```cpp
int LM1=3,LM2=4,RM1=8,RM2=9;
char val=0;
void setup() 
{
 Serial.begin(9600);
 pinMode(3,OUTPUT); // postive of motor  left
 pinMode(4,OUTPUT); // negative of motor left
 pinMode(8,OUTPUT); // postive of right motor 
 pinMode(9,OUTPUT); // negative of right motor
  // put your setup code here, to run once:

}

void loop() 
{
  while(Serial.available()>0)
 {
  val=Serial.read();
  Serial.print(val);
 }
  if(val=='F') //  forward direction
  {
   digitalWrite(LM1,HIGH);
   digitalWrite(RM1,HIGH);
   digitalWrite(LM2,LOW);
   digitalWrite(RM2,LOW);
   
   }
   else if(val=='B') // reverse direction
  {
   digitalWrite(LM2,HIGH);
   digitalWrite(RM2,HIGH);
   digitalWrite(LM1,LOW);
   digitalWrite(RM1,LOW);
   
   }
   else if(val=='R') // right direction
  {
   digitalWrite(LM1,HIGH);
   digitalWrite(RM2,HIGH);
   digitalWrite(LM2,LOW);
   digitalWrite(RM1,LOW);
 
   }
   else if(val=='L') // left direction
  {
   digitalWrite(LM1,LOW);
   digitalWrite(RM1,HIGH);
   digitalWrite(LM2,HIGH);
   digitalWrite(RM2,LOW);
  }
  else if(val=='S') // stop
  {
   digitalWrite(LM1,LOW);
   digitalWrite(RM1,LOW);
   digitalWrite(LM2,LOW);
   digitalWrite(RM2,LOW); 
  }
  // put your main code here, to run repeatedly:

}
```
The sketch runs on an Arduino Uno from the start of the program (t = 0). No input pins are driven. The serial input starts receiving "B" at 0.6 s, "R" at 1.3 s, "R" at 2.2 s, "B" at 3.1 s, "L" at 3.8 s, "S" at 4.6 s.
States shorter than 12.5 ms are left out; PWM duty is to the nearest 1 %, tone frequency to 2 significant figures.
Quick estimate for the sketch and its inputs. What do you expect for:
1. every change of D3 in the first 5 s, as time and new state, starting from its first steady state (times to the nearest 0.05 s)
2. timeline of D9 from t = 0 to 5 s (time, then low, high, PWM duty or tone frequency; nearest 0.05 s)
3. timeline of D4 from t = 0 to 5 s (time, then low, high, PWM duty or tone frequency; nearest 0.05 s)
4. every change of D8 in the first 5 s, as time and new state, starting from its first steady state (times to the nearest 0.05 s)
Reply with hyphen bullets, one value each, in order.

- 0 s low; 1.3 s high; 3.1 s low
- 0 s low; 0.6 s high; 3.8 s low
- 0 s low; 0.6 s high; 1.3 s low; 3.1 s high; 4.6 s low
- 0 s low; 3.8 s high; 4.6 s low
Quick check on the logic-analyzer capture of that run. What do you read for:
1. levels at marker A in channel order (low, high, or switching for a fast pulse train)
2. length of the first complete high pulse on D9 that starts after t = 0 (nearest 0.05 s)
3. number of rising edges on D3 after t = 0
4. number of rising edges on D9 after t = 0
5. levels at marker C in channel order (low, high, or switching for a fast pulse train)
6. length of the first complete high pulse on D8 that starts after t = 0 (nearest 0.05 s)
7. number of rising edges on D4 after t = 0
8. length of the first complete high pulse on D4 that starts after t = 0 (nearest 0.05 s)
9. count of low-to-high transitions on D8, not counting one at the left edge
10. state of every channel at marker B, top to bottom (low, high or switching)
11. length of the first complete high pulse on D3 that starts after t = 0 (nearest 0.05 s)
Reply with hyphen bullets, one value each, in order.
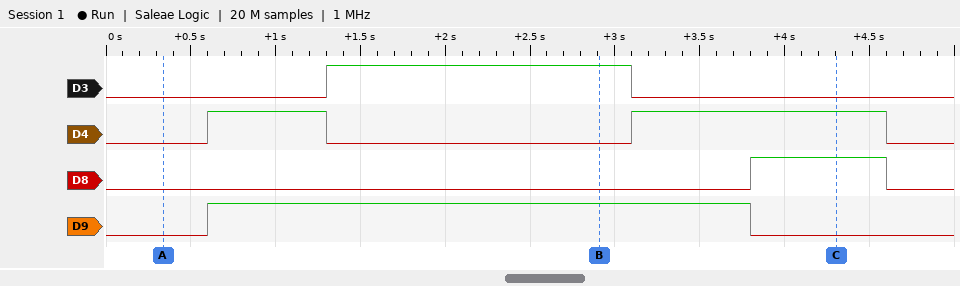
- D3 low, D4 low, D8 low, D9 low
- 3.20 s
- 1
- 1
- D3 low, D4 high, D8 high, D9 low
- 0.80 s
- 2
- 0.70 s
- 1
- D3 high, D4 low, D8 low, D9 high
- 1.80 s
